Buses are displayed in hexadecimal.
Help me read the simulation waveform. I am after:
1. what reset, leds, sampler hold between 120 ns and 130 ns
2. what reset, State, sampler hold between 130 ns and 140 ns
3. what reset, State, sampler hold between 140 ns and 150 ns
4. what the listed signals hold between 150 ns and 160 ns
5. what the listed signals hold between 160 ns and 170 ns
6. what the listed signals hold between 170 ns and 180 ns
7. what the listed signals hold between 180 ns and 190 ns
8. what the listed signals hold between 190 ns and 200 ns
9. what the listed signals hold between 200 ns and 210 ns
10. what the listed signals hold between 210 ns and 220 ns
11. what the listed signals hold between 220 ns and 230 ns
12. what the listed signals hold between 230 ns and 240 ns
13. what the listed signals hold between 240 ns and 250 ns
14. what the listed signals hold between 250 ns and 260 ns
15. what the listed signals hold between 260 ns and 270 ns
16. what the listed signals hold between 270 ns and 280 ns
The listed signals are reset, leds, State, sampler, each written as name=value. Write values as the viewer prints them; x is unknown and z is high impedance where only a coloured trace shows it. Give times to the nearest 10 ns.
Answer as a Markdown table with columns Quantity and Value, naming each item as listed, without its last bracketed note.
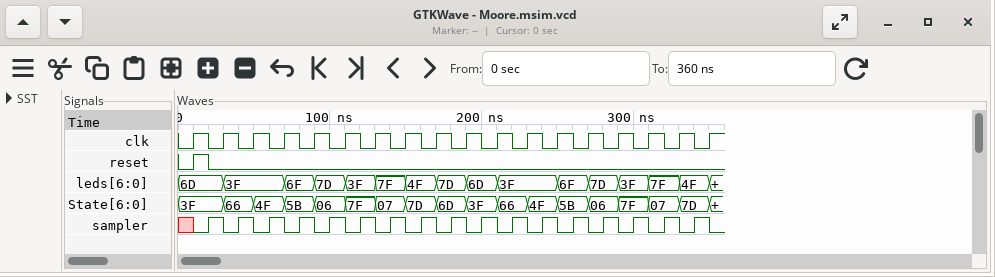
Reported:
| Quantity | Value |
|---|---|
| what reset, leds, sampler hold between 120 ns and 130 ns | reset=0, leds=3F, sampler=1 |
| what reset, State, sampler hold between 130 ns and 140 ns | reset=0, State=07, sampler=0 |
| what reset, State, sampler hold between 140 ns and 150 ns | reset=0, State=07, sampler=1 |
| what the listed signals hold between 150 ns and 160 ns | reset=0, leds=4F, State=7D, sampler=0 |
| what the listed signals hold between 160 ns and 170 ns | reset=0, leds=4F, State=7D, sampler=1 |
| what the listed signals hold between 170 ns and 180 ns | reset=0, leds=7D, State=6D, sampler=0 |
| what the listed signals hold between 180 ns and 190 ns | reset=0, leds=7D, State=6D, sampler=1 |
| what the listed signals hold between 190 ns and 200 ns | reset=0, leds=6D, State=3F, sampler=0 |
| what the listed signals hold between 200 ns and 210 ns | reset=0, leds=6D, State=3F, sampler=1 |
| what the listed signals hold between 210 ns and 220 ns | reset=0, leds=3F, State=66, sampler=0 |
| what the listed signals hold between 220 ns and 230 ns | reset=0, leds=3F, State=66, sampler=1 |
| what the listed signals hold between 230 ns and 240 ns | reset=0, leds=3F, State=4F, sampler=0 |
| what the listed signals hold between 240 ns and 250 ns | reset=0, leds=3F, State=4F, sampler=1 |
| what the listed signals hold between 250 ns and 260 ns | reset=0, leds=6F, State=5B, sampler=0 |
| what the listed signals hold between 260 ns and 270 ns | reset=0, leds=6F, State=5B, sampler=1 |
| what the listed signals hold between 270 ns and 280 ns | reset=0, leds=7D, State=06, sampler=0 |
